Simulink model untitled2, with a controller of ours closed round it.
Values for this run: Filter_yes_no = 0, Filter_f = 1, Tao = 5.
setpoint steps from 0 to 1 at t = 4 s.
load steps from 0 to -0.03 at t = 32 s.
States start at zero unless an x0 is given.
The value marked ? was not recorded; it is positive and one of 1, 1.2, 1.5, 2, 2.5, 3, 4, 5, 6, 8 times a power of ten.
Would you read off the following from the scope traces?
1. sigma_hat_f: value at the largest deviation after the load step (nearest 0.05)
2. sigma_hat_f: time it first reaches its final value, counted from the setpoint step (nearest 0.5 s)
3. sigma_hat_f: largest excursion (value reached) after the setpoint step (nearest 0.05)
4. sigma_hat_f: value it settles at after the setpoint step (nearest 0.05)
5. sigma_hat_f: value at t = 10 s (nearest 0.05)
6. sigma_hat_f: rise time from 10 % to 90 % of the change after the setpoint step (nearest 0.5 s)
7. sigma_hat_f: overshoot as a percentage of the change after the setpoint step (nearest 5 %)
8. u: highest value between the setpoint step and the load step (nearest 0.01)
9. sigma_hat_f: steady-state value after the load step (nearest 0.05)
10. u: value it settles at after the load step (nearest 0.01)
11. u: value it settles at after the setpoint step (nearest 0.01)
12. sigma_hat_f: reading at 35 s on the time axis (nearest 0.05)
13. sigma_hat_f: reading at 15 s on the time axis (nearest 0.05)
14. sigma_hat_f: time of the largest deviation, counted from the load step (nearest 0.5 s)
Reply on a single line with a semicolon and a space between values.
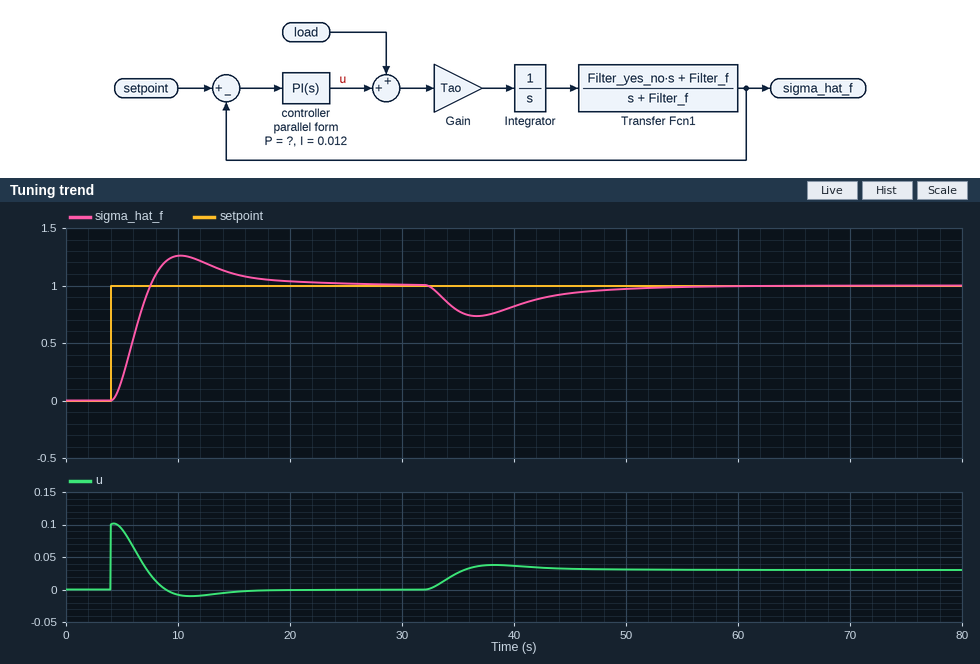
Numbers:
0.75; 3.5 s; 1.25; 1.00; 1.25; 2.5 s; 25 %; 0.10; 1.00; 0.03; 0.00; 0.80; 1.10; 4.5 s
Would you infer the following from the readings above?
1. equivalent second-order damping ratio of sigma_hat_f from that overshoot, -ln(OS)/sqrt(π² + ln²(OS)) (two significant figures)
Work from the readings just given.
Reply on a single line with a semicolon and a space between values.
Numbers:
0.40
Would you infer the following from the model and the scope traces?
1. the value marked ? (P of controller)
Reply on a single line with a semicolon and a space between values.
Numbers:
0.1
